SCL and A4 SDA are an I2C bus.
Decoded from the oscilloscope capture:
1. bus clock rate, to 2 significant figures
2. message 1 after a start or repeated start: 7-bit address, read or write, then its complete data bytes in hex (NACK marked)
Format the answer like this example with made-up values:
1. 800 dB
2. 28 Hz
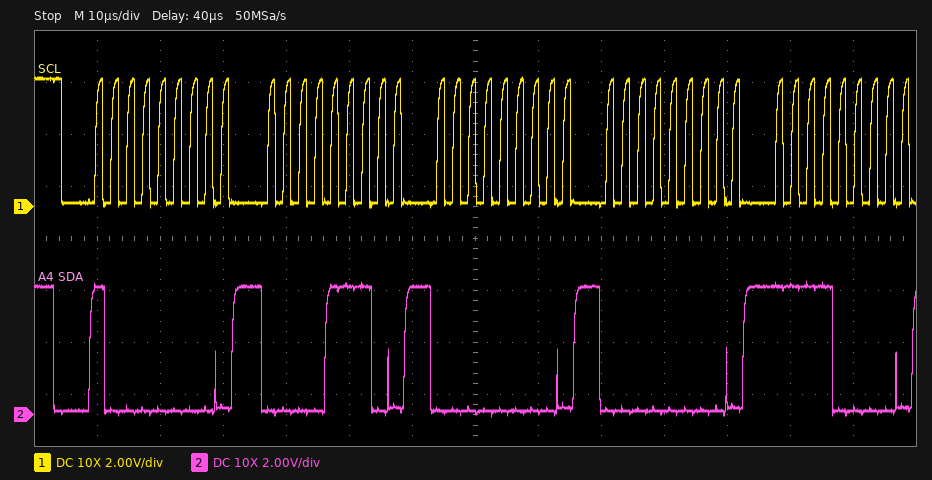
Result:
1. 400 kHz
2. 0x40 write: 0E 00 00 F0
